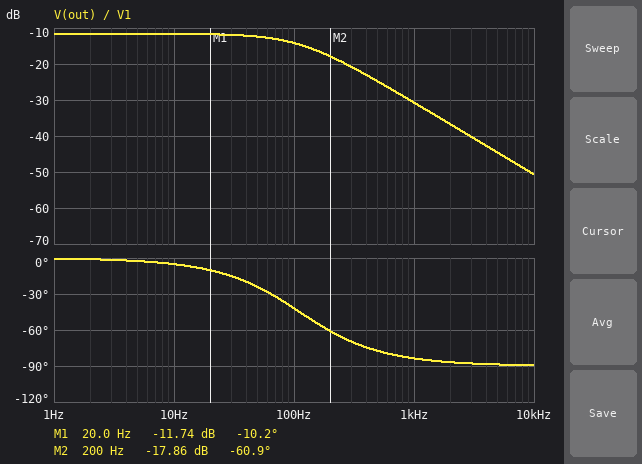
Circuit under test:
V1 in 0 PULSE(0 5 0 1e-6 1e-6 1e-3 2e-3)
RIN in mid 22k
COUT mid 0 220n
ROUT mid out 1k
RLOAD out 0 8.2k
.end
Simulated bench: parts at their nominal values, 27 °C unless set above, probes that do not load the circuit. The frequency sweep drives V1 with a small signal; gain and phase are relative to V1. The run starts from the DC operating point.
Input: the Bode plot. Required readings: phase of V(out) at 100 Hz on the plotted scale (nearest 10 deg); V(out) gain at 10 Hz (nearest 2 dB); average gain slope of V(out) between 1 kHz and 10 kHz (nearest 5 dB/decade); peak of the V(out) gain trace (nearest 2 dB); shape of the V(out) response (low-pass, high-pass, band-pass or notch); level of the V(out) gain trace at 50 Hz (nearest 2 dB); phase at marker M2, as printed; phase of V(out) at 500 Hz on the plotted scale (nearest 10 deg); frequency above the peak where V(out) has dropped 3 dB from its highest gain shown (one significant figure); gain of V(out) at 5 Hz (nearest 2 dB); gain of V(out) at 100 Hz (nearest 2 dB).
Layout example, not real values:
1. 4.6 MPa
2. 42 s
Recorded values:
1. -40 deg
2. -12 dB
3. -20 dB/decade
4. -12 dB
5. low-pass
6. -12 dB
7. -60.9 deg
8. -80 deg
9. 100 Hz
10. -12 dB
11. -14 dB
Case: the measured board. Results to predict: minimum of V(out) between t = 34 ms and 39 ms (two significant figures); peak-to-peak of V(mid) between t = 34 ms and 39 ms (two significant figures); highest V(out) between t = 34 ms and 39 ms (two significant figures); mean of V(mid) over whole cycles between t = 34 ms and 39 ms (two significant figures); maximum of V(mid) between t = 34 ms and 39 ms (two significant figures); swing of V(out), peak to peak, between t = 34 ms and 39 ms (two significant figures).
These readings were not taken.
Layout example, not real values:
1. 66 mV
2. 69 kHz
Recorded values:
1. 440 mV
2. 500 mV
3. 880 mV
4. 740 mV
5. 990 mV
6. 440 mV
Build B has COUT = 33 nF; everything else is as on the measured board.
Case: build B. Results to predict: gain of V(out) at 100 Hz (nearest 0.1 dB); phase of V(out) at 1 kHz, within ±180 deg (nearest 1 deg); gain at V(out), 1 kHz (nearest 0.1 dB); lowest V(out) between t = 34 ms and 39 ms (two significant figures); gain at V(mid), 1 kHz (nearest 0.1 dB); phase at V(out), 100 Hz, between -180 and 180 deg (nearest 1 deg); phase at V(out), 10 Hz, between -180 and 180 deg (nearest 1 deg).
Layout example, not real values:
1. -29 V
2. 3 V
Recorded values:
1. -11.7 dB
2. -53 deg
3. -16.1 dB
4. 12 mV
5. -15.1 dB
6. -8 deg
7. -1 deg
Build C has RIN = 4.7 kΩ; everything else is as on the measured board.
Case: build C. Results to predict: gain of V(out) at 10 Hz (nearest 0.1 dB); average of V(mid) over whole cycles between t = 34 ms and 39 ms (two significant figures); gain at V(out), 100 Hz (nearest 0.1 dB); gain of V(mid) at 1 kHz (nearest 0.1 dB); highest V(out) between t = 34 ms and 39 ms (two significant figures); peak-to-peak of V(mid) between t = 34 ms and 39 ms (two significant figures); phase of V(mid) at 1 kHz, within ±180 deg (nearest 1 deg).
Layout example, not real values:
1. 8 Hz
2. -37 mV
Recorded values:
1. -4.6 dB
2. 1.7 V
3. -5.3 dB
4. -16.5 dB
5. 2.4 V
6. 2.1 V
7. -77 deg
